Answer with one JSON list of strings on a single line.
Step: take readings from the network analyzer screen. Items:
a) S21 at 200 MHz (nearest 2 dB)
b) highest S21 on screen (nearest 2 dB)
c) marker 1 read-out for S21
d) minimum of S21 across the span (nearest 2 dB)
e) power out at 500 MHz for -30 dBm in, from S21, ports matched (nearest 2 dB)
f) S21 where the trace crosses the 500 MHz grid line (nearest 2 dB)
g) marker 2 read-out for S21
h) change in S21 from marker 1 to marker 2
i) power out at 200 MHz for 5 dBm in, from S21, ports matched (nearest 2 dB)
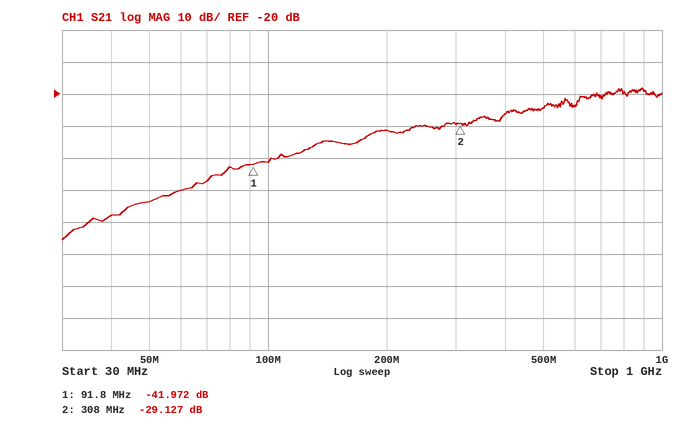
["-32 dB", "-18 dB", "-41.972 dB", "-66 dB", "-54 dBm", "-24 dB", "-29.127 dB", "12.845 dB", "-26 dBm"]
